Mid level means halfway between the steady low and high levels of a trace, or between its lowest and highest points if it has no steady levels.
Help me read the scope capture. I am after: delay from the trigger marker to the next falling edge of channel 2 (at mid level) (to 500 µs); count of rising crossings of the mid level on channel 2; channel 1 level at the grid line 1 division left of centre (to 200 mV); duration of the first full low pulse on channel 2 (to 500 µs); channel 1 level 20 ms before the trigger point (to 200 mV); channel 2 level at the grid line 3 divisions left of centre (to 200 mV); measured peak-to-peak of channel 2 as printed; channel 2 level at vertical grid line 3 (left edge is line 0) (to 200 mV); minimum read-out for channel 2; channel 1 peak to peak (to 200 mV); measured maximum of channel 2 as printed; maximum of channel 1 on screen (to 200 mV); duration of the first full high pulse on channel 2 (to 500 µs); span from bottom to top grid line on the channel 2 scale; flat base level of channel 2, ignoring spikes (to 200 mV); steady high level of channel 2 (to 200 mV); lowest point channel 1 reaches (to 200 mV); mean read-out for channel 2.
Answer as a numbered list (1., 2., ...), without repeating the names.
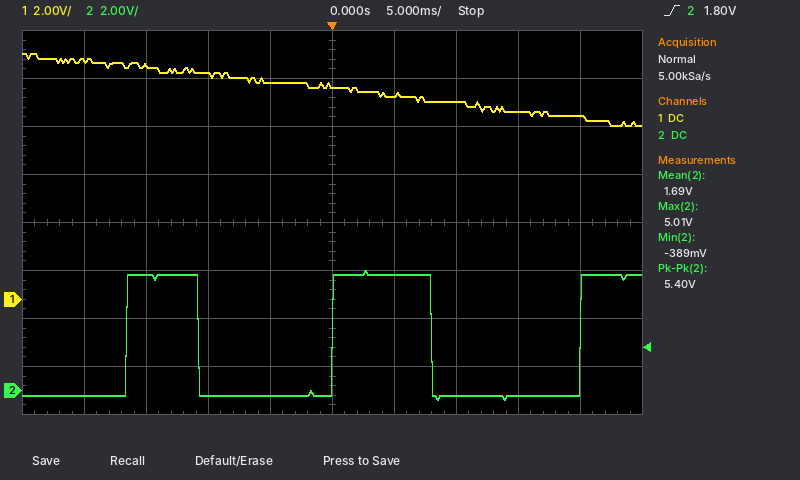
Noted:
1. 8.0 ms
2. 3
3. 9.0 V
4. 11.0 ms
5. 10.0 V
6. 4.8 V
7. 5.40 V
8. -200 mV
9. -389 mV
10. 3.0 V
11. 5.01 V
12. 10.2 V
13. 6.0 ms
14. 16 V
15. -200 mV
16. 4.8 V
17. 7.2 V
18. 1.69 V
